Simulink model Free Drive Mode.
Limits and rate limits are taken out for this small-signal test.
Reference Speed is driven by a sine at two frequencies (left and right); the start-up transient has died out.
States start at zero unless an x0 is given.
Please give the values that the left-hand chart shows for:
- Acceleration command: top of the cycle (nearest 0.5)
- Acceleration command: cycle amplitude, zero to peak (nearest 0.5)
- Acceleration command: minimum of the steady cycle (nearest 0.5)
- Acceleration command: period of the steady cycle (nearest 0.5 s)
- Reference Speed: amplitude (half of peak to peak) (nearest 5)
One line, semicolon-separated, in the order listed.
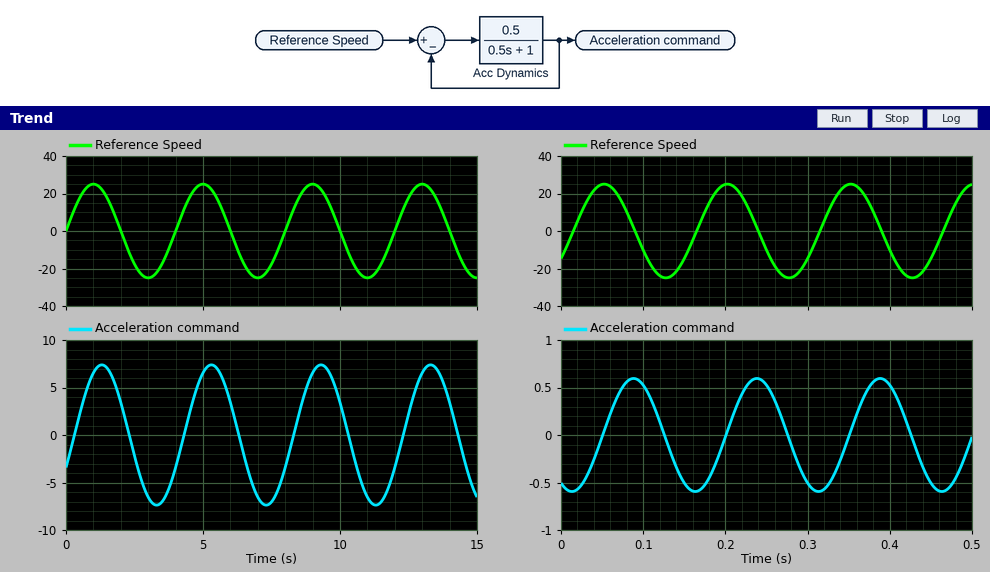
7.5; 7.5; -7.5; 4.0 s; 25
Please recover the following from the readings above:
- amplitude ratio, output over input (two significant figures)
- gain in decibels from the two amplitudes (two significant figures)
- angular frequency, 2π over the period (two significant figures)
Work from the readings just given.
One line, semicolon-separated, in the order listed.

0.30; -10 dB; 1.6 rad/s
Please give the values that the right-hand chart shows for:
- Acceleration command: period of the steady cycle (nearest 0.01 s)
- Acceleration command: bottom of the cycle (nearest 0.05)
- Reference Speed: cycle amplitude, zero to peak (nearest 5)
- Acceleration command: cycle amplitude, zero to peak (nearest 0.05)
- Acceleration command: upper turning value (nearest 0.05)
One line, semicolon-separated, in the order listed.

0.15 s; -0.60; 25; 0.60; 0.60
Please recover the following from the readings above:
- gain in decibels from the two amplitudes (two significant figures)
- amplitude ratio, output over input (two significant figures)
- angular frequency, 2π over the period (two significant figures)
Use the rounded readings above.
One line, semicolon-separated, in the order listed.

-32 dB; 0.024; 42 rad/s
